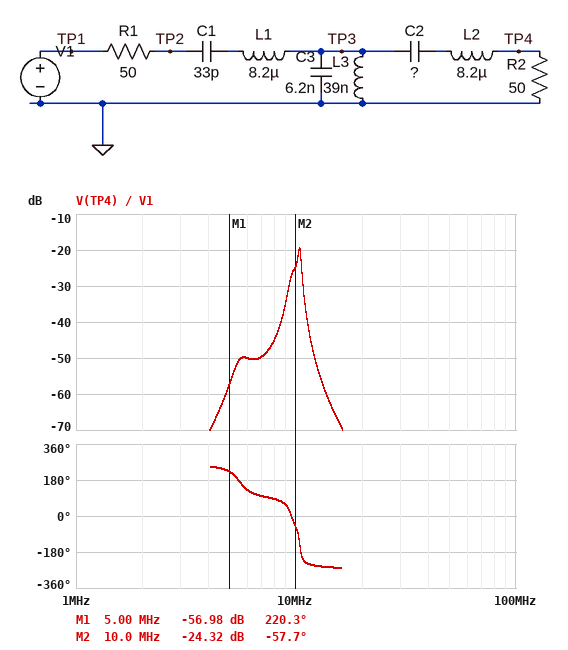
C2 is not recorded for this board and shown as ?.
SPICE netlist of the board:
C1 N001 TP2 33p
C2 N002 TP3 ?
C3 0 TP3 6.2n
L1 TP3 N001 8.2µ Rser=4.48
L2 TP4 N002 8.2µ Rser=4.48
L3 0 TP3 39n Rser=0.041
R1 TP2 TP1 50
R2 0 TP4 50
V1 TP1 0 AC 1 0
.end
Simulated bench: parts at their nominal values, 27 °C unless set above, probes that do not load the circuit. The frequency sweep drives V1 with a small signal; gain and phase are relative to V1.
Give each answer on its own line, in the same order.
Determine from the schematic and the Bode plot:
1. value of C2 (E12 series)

100 pF
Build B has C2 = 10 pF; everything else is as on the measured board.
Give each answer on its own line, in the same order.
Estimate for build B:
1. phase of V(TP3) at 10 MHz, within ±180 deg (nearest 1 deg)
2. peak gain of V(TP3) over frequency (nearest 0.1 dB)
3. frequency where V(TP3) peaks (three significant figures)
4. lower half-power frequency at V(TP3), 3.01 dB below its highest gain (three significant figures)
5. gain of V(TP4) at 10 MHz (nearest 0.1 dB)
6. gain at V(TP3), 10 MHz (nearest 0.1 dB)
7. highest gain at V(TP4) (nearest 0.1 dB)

20 deg
-1.5 dB
10.3 MHz
10.1 MHz
-33.0 dB
-6.4 dB
-27.6 dB
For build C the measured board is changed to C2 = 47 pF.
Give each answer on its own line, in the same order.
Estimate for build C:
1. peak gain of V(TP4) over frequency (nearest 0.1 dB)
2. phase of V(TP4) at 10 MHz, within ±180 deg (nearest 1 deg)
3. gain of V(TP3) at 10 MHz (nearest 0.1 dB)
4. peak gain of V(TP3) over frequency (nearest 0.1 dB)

-14.9 dB
-49 deg
-7.8 dB
-2.1 dB
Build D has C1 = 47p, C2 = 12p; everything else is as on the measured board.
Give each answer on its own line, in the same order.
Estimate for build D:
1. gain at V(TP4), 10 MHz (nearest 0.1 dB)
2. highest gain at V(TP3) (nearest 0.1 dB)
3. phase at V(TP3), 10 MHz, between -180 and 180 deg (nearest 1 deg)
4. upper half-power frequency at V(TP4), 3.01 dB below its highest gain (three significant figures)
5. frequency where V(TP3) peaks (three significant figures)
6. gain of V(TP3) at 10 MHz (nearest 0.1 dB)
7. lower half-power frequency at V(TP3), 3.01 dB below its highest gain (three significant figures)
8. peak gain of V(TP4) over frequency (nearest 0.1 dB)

-37.1 dB
-4.2 dB
-4 deg
10.4 MHz
10.3 MHz
-12.9 dB
10.2 MHz
-27.9 dB
